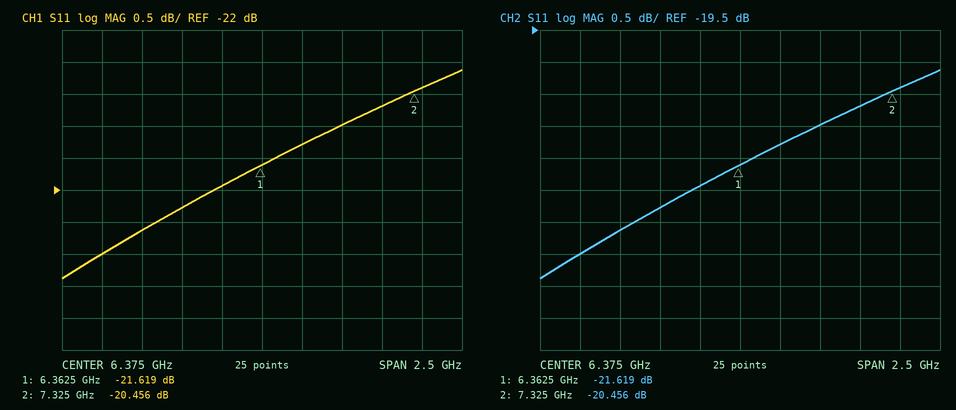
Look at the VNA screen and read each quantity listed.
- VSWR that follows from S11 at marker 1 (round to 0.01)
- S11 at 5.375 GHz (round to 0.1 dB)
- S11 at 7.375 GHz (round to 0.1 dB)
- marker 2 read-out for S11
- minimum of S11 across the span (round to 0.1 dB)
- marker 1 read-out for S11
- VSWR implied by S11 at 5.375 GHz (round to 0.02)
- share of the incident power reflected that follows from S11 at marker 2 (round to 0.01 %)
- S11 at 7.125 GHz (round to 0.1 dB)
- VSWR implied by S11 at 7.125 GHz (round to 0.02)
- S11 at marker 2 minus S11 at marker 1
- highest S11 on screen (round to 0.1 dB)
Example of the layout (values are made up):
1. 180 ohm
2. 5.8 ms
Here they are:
1. 1.18
2. -23.0 dB
3. -20.4 dB
4. -20.456 dB
5. -23.4 dB
6. -21.619 dB
7. 1.16
8. 0.90 %
9. -20.7 dB
10. 1.20
11. 1.163 dB
12. -20.1 dB
